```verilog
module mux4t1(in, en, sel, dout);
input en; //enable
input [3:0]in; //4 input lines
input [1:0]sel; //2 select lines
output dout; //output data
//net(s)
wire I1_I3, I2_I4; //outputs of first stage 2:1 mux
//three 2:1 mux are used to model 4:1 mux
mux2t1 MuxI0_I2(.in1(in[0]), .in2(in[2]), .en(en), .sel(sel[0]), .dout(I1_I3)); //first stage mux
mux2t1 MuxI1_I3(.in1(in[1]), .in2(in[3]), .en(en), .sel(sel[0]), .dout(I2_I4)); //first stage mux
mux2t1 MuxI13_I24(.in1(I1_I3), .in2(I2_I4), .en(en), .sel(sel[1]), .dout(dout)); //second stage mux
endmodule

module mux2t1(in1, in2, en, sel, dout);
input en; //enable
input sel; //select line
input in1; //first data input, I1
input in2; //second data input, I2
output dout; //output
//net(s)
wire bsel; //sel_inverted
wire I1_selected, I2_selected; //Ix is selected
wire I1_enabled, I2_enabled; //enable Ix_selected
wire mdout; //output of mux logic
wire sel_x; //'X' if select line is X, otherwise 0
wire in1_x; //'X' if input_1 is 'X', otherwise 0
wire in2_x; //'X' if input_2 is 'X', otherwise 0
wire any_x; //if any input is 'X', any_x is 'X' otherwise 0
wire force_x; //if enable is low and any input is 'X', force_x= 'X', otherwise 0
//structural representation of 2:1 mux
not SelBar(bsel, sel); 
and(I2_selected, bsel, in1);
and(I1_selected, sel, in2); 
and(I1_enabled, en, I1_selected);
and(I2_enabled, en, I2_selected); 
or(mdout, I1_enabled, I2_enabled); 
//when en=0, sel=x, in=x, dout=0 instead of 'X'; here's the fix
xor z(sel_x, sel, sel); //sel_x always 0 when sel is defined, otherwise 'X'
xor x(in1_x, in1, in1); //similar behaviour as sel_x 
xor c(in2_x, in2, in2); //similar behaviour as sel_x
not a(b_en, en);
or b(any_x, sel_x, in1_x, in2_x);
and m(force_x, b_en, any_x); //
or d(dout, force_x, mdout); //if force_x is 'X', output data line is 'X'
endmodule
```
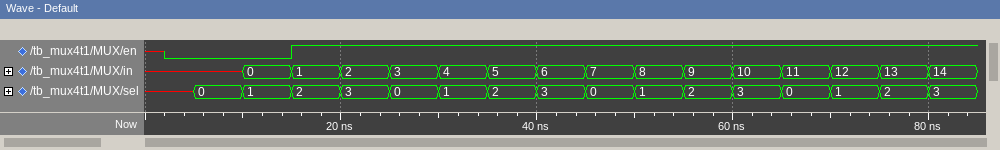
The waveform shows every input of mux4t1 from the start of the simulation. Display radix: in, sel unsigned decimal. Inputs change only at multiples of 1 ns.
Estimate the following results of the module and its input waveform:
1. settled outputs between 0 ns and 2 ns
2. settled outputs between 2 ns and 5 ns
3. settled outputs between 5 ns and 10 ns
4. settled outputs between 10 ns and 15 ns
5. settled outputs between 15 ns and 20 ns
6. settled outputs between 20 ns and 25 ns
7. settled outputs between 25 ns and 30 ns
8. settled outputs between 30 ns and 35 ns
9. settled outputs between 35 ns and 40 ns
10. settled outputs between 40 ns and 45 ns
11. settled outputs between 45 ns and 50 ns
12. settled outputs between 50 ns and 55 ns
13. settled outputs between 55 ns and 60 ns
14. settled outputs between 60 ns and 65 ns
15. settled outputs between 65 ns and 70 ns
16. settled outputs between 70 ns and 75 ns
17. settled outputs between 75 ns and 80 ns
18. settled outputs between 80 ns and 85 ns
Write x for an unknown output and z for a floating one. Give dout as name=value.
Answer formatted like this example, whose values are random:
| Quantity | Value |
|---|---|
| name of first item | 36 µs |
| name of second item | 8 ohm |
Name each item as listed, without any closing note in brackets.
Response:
| Quantity | Value |
|---|---|
| settled outputs between 0 ns and 2 ns | dout=x |
| settled outputs between 2 ns and 5 ns | dout=x |
| settled outputs between 5 ns and 10 ns | dout=x |
| settled outputs between 10 ns and 15 ns | dout=0 |
| settled outputs between 15 ns and 20 ns | dout=0 |
| settled outputs between 20 ns and 25 ns | dout=0 |
| settled outputs between 25 ns and 30 ns | dout=1 |
| settled outputs between 30 ns and 35 ns | dout=1 |
| settled outputs between 35 ns and 40 ns | dout=0 |
| settled outputs between 40 ns and 45 ns | dout=0 |
| settled outputs between 45 ns and 50 ns | dout=1 |
| settled outputs between 50 ns and 55 ns | dout=0 |
| settled outputs between 55 ns and 60 ns | dout=0 |
| settled outputs between 60 ns and 65 ns | dout=1 |
| settled outputs between 65 ns and 70 ns | dout=1 |
| settled outputs between 70 ns and 75 ns | dout=1 |
| settled outputs between 75 ns and 80 ns | dout=0 |
| settled outputs between 80 ns and 85 ns | dout=1 |
